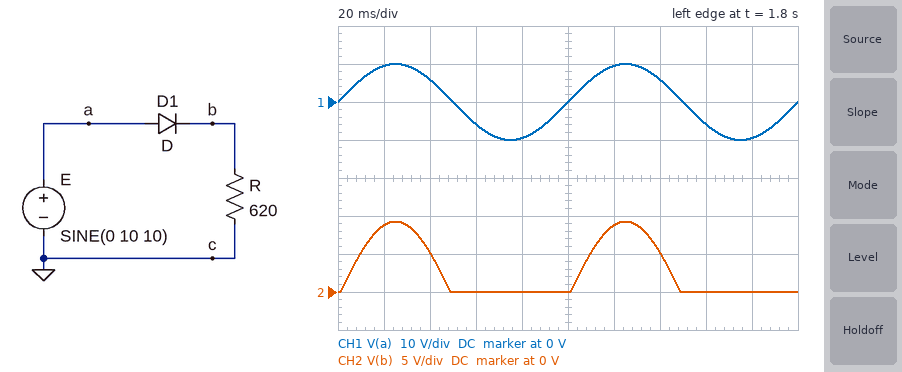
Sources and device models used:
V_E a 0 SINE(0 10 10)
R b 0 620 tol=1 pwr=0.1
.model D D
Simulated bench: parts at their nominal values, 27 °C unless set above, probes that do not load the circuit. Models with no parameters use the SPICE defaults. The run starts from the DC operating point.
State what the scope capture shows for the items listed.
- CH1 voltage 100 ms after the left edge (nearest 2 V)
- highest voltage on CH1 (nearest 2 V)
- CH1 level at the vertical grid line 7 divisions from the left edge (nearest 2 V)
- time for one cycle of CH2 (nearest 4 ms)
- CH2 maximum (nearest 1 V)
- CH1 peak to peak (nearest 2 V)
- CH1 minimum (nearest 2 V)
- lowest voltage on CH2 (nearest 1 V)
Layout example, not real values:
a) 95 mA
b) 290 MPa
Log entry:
a) 0 V
b) 10 V
c) 6 V
d) 100 ms
e) 9 V
f) 20 V
g) -10 V
h) 0 V
